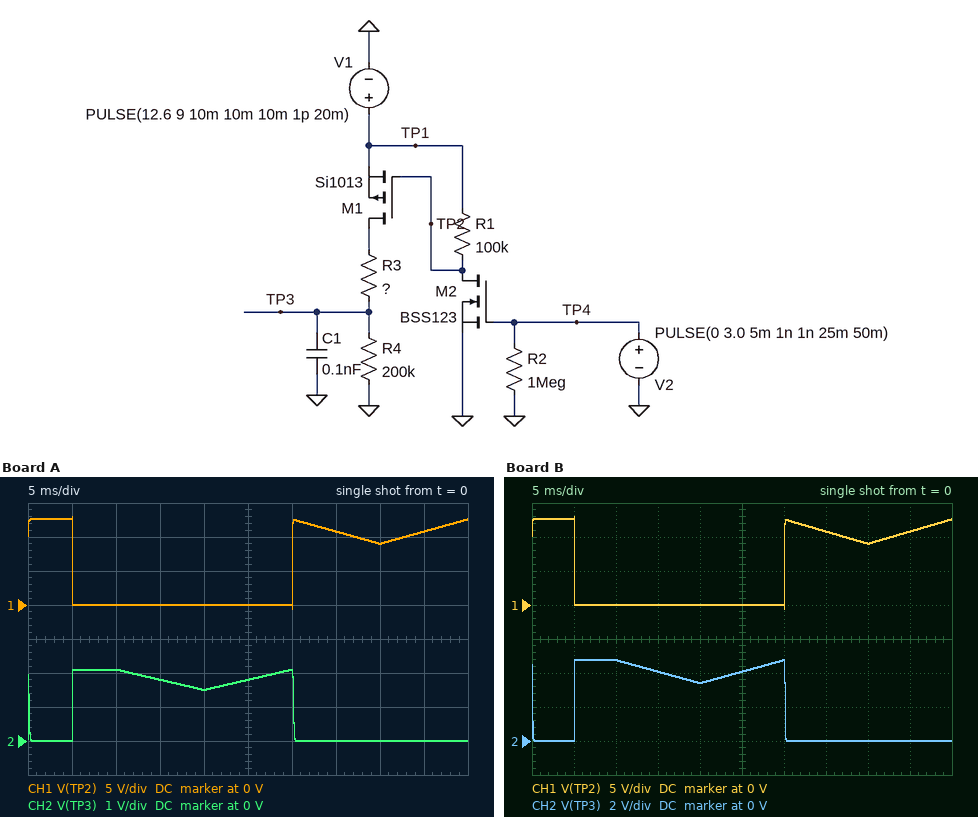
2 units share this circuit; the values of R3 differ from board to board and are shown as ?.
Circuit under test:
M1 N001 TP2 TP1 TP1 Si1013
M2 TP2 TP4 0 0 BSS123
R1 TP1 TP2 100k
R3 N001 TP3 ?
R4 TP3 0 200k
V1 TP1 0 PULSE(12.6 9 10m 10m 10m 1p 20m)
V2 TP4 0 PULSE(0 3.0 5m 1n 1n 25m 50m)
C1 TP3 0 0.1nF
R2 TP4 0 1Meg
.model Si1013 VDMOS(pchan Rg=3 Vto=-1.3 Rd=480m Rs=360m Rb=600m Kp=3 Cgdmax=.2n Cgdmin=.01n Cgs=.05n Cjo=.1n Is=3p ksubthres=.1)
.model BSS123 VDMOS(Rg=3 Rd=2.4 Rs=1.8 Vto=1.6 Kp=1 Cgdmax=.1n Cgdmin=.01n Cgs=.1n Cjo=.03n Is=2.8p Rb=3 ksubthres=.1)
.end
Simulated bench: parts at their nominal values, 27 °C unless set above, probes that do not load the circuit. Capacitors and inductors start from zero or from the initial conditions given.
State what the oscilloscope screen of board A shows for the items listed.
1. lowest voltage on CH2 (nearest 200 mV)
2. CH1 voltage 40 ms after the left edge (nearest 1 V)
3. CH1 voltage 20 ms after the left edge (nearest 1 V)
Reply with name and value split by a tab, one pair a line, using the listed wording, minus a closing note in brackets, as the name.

lowest voltage on CH2	0 V
CH1 voltage 40 ms after the left edge	9 V
CH1 voltage 20 ms after the left edge	0 V
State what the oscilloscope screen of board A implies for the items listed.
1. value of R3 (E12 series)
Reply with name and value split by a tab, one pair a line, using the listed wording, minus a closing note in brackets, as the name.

value of R3	1 MΩ
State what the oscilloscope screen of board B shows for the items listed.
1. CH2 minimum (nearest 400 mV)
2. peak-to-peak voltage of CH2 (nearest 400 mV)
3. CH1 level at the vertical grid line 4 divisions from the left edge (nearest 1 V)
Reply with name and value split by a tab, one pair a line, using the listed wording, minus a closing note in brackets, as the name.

CH2 minimum	0 V
peak-to-peak voltage of CH2	4.8 V
CH1 level at the vertical grid line 4 divisions from the left edge	0 V
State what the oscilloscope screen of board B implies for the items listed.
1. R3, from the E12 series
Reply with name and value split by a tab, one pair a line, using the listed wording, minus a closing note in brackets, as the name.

R3, from the E12 series	330 kΩ
